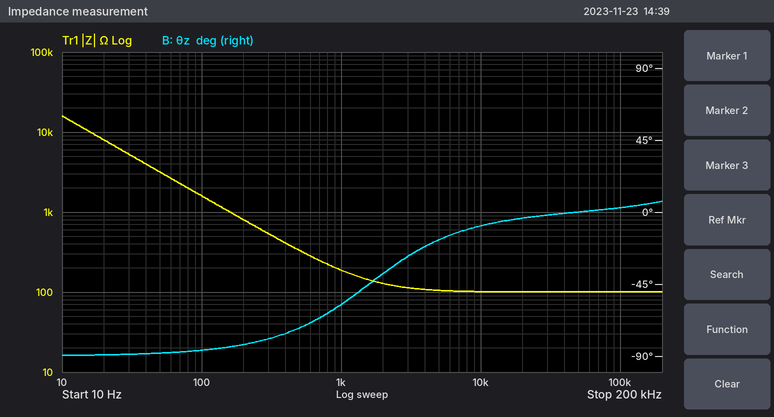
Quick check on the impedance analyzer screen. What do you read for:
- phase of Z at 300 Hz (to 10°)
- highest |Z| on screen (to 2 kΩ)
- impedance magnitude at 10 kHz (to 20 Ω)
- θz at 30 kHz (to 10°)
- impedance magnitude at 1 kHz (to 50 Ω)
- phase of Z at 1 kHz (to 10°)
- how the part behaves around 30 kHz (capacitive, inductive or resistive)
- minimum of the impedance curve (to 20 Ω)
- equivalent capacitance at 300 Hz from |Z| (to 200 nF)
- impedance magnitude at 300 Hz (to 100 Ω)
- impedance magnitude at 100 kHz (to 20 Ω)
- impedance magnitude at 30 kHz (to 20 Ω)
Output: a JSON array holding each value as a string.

["-80°", "16 kΩ", "100 Ω", "0°", "200 Ω", "-60°", "resistive", "100 Ω", "1.0 µF", "500 Ω", "100 Ω", "100 Ω"]
